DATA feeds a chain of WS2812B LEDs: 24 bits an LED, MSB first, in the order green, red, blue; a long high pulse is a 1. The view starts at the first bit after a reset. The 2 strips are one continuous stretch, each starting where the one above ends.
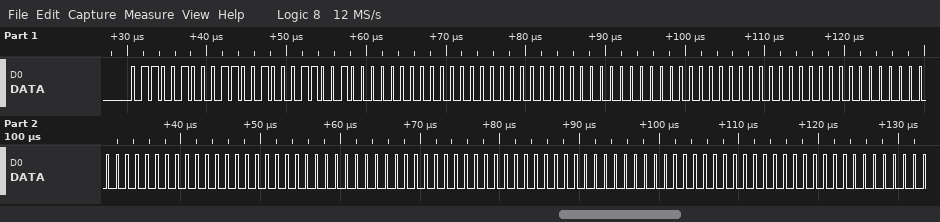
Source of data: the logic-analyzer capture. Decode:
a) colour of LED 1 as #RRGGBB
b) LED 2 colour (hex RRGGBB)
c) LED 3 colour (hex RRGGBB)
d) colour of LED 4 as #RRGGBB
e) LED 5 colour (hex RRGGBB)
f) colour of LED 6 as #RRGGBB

#646464
#000000
#000000
#000000
#000000
#000000
